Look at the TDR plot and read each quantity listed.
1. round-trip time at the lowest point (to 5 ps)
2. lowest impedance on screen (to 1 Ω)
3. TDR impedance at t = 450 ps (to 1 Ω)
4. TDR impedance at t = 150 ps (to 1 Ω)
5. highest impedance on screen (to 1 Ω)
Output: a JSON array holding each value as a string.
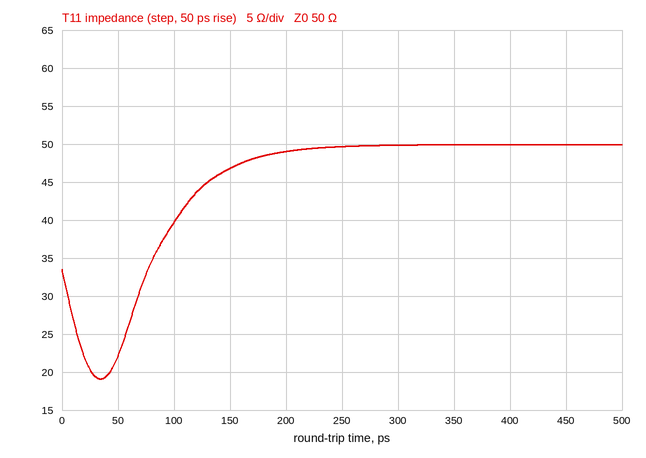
["35 ps", "19 Ω", "50 Ω", "47 Ω", "50 Ω"]
